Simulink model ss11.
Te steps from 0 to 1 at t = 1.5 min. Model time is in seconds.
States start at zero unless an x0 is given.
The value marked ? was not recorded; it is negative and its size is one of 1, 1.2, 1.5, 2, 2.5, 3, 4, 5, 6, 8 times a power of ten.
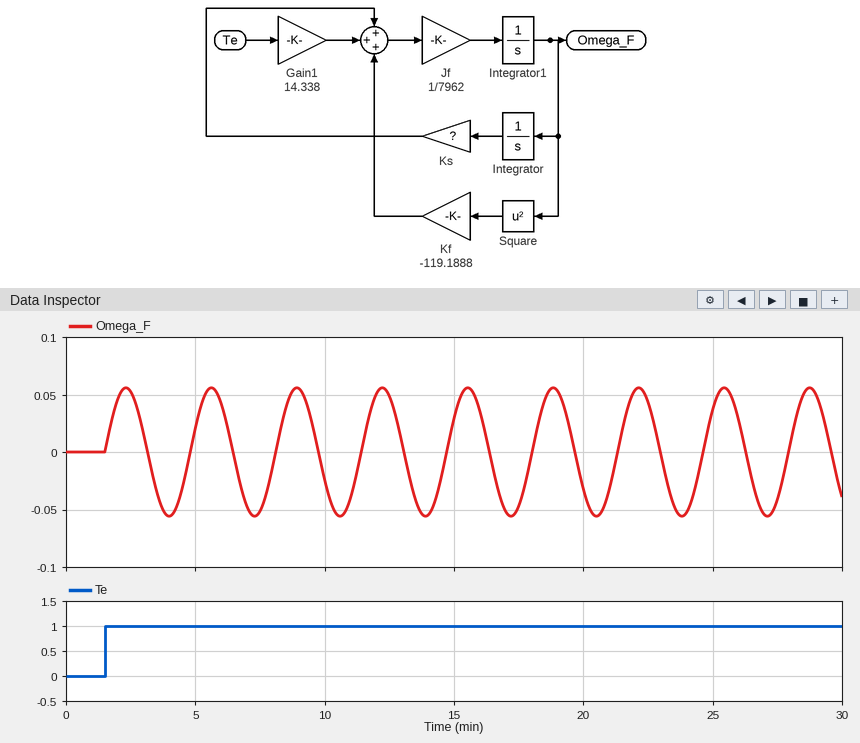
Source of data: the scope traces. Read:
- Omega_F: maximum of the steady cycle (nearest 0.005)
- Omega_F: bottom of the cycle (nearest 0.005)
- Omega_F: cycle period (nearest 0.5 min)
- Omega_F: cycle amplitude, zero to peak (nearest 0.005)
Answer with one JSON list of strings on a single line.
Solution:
["0.055", "-0.055", "3.5 min", "0.055"]
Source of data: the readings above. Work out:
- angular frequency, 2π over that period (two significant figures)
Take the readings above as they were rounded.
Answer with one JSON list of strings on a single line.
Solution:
["1.8 rad/min"]
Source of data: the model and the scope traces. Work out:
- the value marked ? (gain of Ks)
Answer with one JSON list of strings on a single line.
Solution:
["-8"]
